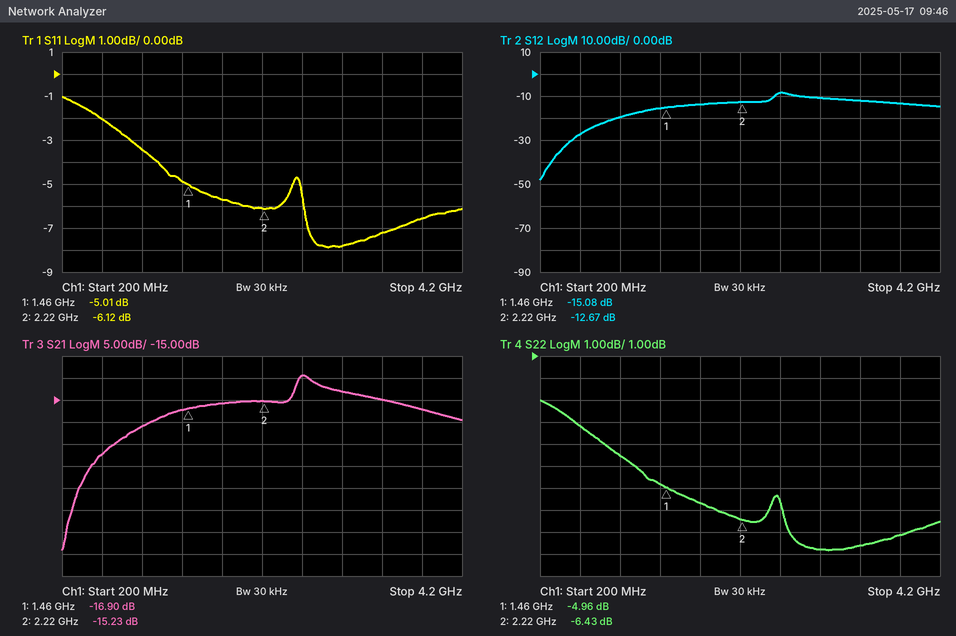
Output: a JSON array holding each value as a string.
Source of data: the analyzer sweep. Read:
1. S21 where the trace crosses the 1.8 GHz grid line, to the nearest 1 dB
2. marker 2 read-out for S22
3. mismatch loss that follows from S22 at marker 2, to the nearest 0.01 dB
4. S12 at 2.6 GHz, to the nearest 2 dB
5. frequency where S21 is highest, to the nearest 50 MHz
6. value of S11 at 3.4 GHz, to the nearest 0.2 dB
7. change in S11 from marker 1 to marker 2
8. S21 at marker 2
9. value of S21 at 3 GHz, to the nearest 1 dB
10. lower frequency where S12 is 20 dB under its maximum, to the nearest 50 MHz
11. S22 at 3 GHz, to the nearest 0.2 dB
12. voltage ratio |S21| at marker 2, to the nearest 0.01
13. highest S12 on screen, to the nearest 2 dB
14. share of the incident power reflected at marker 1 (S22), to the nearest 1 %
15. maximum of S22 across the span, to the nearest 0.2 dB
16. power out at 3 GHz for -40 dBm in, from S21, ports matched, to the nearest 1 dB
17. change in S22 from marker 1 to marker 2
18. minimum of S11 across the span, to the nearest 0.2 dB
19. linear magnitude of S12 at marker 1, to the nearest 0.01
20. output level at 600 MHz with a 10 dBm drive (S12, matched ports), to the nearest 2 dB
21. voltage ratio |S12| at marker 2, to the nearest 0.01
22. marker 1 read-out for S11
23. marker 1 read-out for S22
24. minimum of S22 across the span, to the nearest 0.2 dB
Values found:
["-16 dB", "-6.43 dB", "1.12 dB", "-8 dB", "2.60 GHz", "-7.2 dB", "-1.11 dB", "-15.23 dB", "-13 dB", "550 MHz", "-7.8 dB", "0.17", "-8 dB", "32 %", "-1.0 dB", "-53 dBm", "-1.47 dB", "-7.8 dB", "0.18", "-18 dBm", "0.23", "-5.01 dB", "-4.96 dB", "-7.8 dB"]
